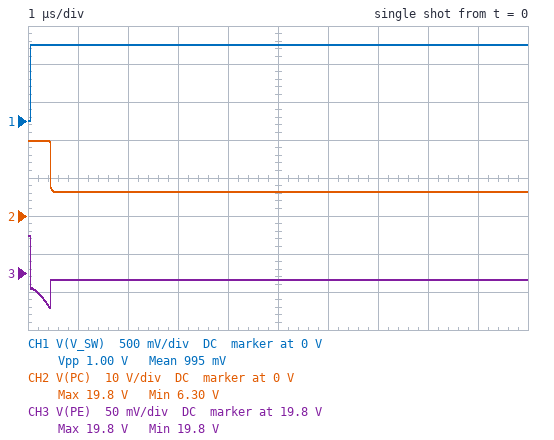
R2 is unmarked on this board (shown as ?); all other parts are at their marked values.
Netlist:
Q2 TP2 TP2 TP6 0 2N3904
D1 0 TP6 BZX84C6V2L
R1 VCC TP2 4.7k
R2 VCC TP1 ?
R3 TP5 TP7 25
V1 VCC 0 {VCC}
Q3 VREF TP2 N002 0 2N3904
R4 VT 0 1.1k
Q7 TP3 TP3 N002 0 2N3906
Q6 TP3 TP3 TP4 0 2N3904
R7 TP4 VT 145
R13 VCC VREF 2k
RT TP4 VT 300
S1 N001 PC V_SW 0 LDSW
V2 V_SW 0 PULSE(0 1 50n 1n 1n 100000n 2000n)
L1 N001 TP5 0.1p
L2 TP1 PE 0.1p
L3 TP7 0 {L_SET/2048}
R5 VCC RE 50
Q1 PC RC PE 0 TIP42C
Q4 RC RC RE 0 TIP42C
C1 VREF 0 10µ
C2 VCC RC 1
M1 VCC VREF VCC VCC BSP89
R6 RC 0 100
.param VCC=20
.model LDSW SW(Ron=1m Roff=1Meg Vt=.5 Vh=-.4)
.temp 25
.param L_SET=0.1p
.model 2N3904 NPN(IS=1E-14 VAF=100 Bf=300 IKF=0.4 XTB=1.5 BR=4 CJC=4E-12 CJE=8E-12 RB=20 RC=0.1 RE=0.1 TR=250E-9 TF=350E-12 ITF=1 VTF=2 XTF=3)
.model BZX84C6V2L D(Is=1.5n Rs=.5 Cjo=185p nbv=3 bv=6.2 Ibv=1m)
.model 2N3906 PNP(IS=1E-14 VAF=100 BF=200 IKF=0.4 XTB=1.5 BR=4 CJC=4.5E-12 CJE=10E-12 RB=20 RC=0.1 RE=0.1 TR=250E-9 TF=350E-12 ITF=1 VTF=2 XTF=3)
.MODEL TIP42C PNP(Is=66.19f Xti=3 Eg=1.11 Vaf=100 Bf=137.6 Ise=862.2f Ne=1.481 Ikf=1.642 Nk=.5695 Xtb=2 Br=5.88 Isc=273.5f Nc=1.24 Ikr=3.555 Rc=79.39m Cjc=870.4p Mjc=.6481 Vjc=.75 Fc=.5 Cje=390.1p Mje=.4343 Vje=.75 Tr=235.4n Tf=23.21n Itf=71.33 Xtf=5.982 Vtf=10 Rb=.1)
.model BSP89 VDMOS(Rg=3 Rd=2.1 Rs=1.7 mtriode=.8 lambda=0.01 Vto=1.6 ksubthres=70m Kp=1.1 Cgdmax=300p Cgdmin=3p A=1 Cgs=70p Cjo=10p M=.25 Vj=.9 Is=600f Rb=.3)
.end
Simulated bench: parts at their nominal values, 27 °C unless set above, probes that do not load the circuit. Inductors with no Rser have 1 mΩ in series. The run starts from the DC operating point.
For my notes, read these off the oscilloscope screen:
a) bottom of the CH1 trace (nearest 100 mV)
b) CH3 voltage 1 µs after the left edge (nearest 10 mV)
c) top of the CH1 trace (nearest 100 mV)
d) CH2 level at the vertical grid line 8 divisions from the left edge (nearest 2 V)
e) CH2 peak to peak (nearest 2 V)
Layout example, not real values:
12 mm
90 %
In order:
0 V
19.79 V
1.0 V
6 V
14 V
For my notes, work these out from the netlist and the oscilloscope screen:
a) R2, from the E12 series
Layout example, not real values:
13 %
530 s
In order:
0.82 Ω
